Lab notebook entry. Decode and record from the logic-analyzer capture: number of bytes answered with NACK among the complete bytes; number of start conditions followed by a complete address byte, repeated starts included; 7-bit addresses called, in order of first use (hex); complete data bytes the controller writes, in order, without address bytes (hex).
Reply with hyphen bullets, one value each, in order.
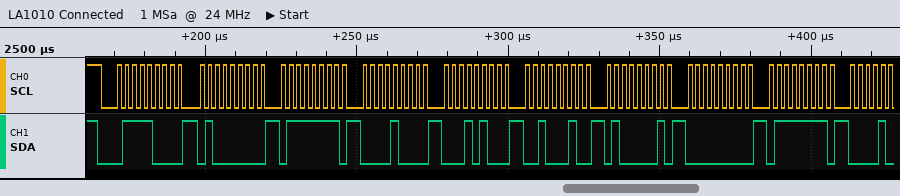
- 0
- 1
- 0x3C
- 40 7F 08 14 22 41 00 7F
